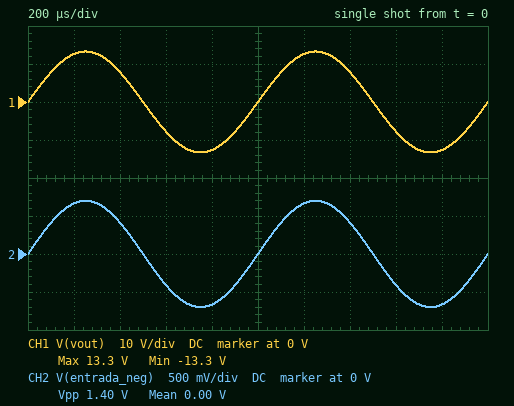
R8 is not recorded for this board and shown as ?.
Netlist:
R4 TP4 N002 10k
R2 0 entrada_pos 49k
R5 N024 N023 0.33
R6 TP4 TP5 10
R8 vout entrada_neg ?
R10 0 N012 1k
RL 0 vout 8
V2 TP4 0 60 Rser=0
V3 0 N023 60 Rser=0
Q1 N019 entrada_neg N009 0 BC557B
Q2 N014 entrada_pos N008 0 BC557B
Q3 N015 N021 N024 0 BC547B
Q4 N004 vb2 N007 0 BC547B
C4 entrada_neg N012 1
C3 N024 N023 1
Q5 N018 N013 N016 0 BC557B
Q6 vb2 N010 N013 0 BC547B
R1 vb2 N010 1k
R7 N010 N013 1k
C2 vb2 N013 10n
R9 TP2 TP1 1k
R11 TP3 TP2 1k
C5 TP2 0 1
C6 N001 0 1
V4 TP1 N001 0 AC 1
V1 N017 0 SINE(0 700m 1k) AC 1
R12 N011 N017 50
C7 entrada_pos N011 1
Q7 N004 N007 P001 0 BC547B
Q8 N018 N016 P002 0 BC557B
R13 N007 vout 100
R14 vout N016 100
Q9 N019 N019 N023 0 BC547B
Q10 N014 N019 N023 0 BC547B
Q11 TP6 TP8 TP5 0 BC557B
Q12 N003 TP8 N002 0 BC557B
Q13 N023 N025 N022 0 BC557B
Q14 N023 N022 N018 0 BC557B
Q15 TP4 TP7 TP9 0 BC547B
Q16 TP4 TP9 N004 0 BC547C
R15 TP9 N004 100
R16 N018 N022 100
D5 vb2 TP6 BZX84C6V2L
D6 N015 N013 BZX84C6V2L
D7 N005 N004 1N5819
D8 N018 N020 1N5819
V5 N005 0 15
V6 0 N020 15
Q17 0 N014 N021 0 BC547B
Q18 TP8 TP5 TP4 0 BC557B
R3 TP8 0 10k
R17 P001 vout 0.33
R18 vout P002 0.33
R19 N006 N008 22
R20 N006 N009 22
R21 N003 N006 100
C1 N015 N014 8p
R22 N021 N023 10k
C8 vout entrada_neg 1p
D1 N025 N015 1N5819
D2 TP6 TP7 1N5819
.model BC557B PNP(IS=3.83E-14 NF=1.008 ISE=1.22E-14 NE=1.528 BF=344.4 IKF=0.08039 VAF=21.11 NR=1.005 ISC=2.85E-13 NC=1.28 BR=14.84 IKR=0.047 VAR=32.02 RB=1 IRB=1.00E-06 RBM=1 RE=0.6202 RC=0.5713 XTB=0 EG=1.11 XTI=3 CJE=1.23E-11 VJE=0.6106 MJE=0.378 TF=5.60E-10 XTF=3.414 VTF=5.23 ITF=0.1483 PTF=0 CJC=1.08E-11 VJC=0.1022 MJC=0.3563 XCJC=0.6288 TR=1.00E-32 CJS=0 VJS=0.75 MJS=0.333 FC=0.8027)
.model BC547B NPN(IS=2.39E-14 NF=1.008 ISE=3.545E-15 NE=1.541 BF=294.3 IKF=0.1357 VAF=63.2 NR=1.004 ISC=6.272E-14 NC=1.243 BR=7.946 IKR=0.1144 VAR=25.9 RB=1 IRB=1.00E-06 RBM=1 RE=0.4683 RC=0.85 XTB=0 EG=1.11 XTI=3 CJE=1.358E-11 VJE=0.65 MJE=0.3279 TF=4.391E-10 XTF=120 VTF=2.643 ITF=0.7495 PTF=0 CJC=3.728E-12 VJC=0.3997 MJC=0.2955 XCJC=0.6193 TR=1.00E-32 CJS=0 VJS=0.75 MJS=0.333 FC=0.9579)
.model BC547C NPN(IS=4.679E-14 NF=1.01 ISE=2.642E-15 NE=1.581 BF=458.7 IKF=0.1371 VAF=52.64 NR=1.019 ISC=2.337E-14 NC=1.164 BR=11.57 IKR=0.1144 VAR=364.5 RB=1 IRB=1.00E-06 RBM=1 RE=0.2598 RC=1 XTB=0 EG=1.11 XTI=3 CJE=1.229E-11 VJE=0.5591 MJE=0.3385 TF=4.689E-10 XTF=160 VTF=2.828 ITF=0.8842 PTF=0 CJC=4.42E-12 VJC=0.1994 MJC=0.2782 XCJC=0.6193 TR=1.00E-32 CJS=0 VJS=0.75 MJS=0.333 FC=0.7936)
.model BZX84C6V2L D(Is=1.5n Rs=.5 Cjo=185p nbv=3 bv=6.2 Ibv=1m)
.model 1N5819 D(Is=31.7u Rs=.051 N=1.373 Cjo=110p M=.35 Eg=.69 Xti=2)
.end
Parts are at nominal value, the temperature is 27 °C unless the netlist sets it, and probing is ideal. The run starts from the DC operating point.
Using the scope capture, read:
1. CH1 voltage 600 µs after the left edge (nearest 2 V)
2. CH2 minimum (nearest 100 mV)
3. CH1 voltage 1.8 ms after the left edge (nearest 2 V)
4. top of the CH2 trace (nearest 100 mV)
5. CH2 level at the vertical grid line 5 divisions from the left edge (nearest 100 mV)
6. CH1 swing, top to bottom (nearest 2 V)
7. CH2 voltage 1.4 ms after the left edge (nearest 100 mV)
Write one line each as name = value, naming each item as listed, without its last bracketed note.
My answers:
CH1 voltage 600 µs after the left edge = -8 V
CH2 minimum = -700 mV
CH1 voltage 1.8 ms after the left edge = -12 V
top of the CH2 trace = 700 mV
CH2 level at the vertical grid line 5 divisions from the left edge = 0 V
CH1 swing, top to bottom = 26 V
CH2 voltage 1.4 ms after the left edge = 400 mV
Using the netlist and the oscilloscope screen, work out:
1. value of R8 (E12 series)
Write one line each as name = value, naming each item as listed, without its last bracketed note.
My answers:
value of R8 = 18 kΩ
